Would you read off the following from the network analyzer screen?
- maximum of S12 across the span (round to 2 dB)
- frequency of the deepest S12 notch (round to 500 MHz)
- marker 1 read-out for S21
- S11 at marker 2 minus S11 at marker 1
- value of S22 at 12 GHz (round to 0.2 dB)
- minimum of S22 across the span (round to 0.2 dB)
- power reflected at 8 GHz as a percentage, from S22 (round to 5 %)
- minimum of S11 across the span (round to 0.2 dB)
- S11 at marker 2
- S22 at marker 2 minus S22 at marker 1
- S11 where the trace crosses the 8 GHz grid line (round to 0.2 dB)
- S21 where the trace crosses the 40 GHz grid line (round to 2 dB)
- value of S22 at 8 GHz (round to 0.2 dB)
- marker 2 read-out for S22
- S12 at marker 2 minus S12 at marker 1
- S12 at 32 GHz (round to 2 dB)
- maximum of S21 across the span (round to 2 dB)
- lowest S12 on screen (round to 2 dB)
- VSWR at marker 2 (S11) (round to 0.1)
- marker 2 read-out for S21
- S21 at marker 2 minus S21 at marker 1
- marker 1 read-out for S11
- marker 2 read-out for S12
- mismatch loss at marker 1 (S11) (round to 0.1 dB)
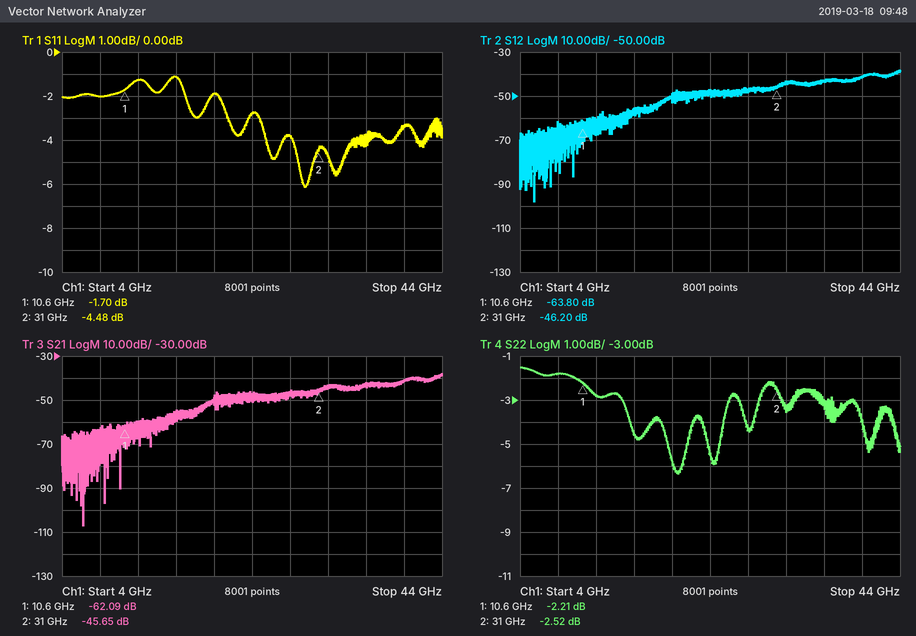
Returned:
-38 dB
5.5 GHz
-62.09 dB
-2.78 dB
-2.8 dB
-6.4 dB
65 %
-6.2 dB
-4.48 dB
-0.31 dB
-2.0 dB
-42 dB
-1.8 dB
-2.52 dB
17.60 dB
-44 dB
-38 dB
-98 dB
4.0
-45.65 dB
16.44 dB
-1.70 dB
-46.20 dB
4.9 dB
